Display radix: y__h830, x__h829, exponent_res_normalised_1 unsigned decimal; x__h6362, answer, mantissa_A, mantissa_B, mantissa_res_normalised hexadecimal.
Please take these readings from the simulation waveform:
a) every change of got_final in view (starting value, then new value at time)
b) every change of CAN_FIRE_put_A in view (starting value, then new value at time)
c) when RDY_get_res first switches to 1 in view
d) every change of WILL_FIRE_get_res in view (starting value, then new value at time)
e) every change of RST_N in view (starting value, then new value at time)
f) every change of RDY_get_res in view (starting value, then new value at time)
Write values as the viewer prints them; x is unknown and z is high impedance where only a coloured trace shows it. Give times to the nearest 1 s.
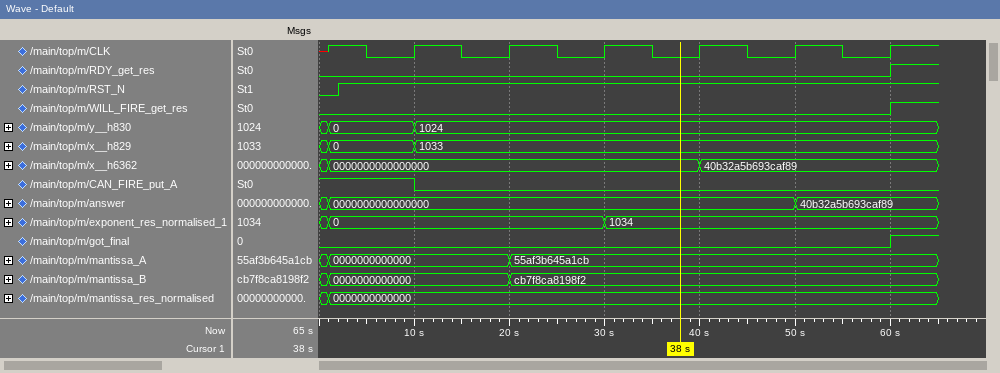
0, 1 at 60 s
1, 0 at 10 s
60 s
0, 1 at 60 s
0, 1 at 2 s
0, 1 at 60 s
